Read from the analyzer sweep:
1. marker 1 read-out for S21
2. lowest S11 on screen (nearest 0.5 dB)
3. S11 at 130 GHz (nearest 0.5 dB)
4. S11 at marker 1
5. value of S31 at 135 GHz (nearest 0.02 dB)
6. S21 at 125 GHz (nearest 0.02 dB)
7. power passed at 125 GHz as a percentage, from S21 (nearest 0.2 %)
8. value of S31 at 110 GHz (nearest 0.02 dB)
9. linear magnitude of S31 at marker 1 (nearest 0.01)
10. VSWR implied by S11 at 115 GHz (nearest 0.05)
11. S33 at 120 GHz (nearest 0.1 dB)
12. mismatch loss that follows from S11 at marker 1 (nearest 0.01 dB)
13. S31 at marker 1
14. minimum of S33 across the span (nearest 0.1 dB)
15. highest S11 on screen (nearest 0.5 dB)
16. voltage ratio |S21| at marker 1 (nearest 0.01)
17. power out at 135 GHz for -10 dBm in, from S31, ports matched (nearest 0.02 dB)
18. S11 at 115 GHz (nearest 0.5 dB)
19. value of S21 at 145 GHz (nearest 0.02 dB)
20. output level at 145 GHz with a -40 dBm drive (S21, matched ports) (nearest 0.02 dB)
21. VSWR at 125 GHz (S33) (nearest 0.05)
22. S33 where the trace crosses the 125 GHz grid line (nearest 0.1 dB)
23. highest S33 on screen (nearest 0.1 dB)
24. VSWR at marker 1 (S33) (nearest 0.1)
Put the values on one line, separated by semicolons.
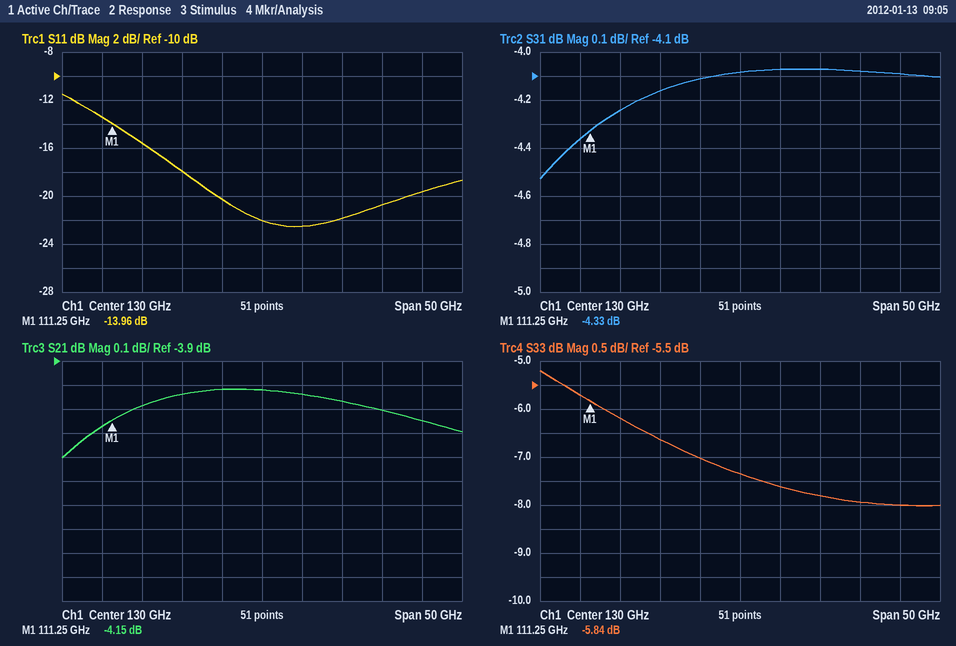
-4.15 dB; -22.5 dB; -22.0 dB; -13.96 dB; -4.08 dB; -4.02 dB; 39.6 %; -4.36 dB; 0.61; 1.40; -6.6 dB; 0.18 dB; -4.33 dB; -8.0 dB; -11.5 dB; 0.62; -14.08 dBm; -15.5 dB; -4.10 dB; -44.10 dBm; 2.60; -7.0 dB; -5.2 dB; 3.1
